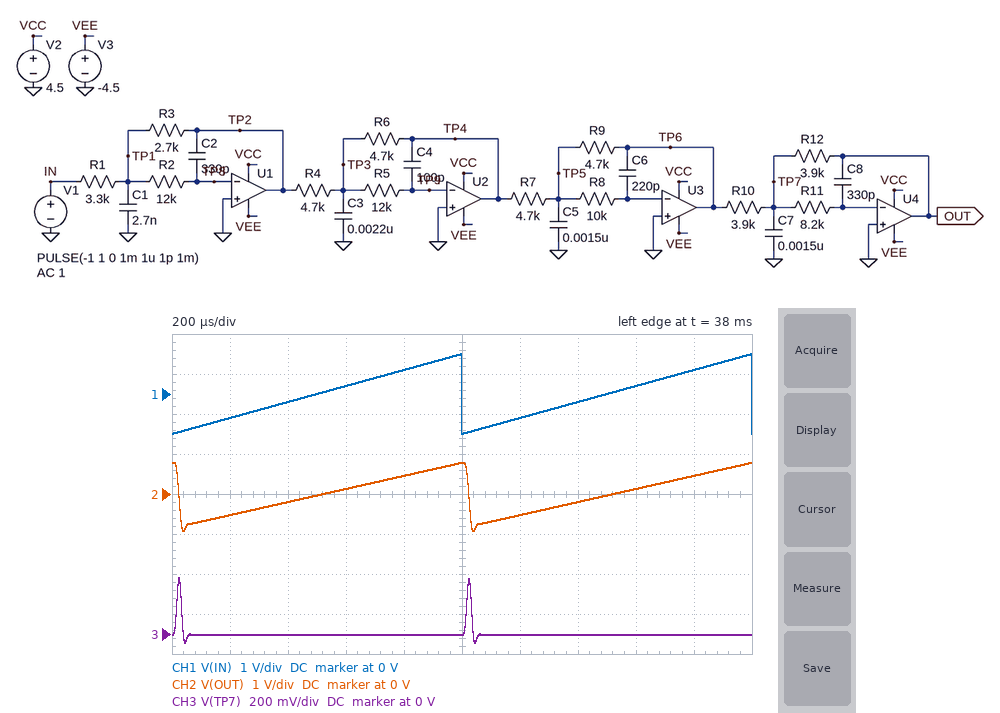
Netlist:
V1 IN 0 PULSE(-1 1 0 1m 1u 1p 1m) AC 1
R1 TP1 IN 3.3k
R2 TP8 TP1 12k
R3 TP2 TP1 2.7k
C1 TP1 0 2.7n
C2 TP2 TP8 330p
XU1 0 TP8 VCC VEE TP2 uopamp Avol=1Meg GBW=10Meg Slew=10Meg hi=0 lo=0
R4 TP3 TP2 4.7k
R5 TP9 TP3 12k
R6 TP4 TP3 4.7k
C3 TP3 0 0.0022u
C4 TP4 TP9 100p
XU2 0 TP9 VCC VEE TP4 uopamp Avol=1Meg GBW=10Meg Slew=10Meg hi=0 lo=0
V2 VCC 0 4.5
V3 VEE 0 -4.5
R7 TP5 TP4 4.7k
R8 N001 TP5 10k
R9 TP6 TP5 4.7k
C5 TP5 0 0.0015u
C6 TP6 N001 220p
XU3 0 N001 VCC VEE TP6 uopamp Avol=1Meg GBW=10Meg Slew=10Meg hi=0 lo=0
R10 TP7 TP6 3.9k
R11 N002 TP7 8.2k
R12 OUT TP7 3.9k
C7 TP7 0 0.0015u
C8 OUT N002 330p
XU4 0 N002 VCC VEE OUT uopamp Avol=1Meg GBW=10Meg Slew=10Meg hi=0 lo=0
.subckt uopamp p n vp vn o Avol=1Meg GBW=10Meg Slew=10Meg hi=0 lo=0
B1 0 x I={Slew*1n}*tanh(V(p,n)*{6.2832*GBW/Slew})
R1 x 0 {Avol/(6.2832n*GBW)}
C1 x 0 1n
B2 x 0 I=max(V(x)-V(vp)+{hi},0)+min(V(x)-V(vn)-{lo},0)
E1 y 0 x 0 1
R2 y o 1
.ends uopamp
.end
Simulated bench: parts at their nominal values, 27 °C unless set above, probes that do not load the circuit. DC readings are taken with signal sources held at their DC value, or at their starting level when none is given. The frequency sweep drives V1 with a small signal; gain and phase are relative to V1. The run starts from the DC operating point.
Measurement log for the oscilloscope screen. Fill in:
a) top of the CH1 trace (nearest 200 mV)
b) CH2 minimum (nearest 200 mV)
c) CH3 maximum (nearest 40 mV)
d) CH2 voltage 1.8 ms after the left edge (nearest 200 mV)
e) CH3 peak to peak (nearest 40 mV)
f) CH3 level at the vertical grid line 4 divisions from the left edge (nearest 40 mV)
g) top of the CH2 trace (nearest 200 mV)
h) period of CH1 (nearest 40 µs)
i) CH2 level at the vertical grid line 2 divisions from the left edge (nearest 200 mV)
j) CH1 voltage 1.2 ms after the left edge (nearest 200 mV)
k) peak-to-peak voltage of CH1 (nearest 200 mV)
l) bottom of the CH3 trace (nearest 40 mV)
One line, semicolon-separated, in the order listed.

1.0 V; -1.0 V; 280 mV; 400 mV; 320 mV; 0 V; 800 mV; 1.00 ms; -200 mV; -600 mV; 2.0 V; -40 mV
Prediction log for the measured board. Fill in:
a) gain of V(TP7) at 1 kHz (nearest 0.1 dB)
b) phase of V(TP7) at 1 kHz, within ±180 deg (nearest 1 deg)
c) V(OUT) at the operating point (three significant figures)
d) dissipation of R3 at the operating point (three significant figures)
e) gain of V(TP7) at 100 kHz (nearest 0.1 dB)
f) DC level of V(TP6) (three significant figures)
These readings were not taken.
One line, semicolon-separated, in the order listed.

-37.1 dB; -98 deg; -818 mV; 248 µW; -63.6 dB; 818 mV
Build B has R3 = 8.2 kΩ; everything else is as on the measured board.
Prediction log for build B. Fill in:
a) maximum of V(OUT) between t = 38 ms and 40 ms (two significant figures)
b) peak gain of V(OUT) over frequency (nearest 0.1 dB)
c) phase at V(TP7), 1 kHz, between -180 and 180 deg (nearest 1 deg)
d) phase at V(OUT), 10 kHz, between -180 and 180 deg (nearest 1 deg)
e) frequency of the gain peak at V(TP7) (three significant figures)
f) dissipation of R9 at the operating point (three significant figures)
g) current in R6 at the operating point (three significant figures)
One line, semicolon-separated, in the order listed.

2.4 V; 7.9 dB; -101 deg; -113 deg; 16.5 kHz; 1.31 mW; 529 µA
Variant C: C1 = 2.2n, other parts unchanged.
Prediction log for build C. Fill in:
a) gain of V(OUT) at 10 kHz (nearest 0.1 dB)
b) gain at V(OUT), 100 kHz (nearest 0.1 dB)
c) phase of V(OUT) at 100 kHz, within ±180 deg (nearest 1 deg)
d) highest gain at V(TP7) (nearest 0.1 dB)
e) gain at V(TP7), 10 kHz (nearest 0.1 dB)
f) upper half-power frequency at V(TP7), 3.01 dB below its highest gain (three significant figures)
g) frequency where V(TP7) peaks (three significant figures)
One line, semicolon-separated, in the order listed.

-2.0 dB; -66.8 dB; 126 deg; -12.2 dB; -17.4 dB; 37.9 kHz; 25.3 kHz
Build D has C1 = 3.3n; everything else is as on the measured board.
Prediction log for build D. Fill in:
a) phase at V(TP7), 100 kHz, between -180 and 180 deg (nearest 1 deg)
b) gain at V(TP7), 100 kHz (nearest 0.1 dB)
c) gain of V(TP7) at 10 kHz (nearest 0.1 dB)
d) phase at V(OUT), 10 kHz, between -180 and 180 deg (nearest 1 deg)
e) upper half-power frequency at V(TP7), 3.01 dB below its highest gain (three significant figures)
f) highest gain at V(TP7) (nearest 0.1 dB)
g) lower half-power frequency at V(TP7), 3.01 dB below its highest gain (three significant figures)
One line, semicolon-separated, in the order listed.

26 deg; -65.2 dB; -17.0 dB; -86 deg; 35.3 kHz; -11.7 dB; 13.2 kHz
